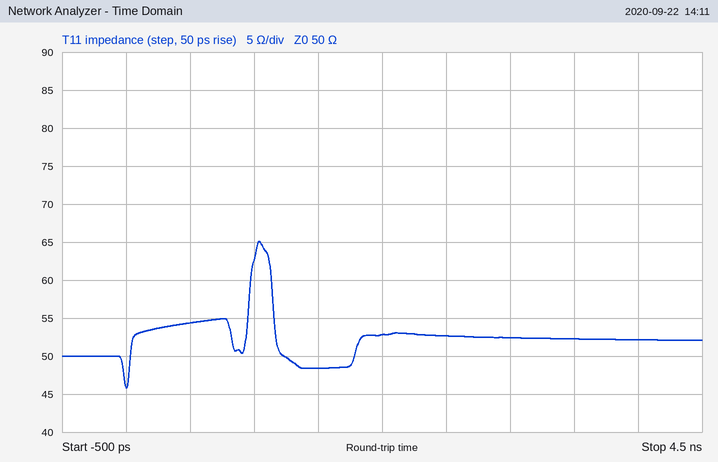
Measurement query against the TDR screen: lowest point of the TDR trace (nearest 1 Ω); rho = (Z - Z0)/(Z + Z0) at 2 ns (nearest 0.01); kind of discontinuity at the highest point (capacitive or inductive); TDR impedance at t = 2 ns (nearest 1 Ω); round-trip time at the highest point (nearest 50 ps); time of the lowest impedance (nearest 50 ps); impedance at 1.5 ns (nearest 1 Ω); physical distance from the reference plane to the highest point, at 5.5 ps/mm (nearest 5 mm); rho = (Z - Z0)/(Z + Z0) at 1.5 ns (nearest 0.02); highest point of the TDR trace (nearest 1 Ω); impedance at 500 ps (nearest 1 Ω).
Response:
46 Ω
+0.03
inductive
53 Ω
1.05 ns
0 ps
48 Ω
95 mm
-0.02
65 Ω
54 Ω
